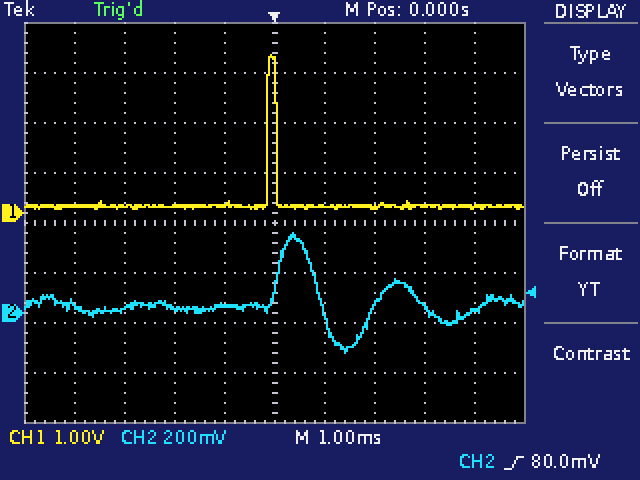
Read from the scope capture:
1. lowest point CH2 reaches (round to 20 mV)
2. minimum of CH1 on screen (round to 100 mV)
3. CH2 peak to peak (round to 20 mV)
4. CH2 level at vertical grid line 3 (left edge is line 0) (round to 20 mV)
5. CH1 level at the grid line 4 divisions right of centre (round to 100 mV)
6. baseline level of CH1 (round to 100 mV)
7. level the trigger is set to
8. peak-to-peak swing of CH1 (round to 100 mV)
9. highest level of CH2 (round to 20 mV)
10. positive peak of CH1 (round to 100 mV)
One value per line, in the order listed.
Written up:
-160 mV
100 mV
480 mV
20 mV
100 mV
100 mV
80.0 mV
3.1 V
320 mV
3.2 V
